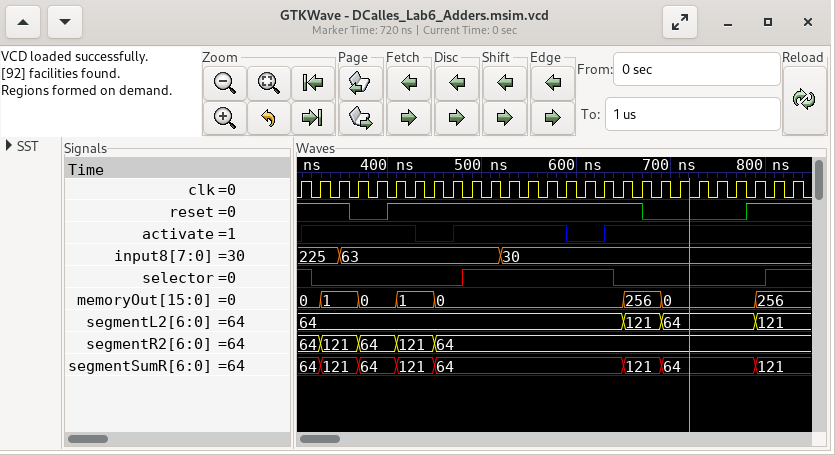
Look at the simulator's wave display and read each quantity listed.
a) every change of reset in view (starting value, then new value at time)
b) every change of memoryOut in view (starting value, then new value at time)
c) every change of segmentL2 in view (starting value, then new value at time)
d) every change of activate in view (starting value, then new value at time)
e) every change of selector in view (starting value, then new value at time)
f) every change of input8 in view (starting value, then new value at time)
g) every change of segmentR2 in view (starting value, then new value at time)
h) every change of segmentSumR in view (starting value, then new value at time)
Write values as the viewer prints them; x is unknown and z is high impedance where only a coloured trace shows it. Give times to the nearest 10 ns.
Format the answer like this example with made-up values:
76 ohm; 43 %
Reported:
1, 0 at 360 ns, 1 at 400 ns, 0 at 670 ns, 1 at 780 ns; 0, 1 at 330 ns, 0 at 370 ns, 1 at 410 ns, 0 at 450 ns, 256 at 650 ns, 0 at 690 ns, 256 at 790 ns; 64, 121 at 650 ns, 64 at 690 ns, 121 at 790 ns; 0, 1 at 310 ns, 0 at 430 ns, 1 at 470 ns, 0 at 590 ns, 1 at 630 ns; 1, 0 at 320 ns, 1 at 480 ns, 0 at 640 ns, 1 at 800 ns; 225, 63 at 350 ns, 30 at 520 ns; 64, 121 at 330 ns, 64 at 370 ns, 121 at 410 ns, 64 at 450 ns; 64, 121 at 330 ns, 64 at 370 ns, 121 at 410 ns, 64 at 450 ns, 121 at 650 ns, 64 at 690 ns, 121 at 790 ns
